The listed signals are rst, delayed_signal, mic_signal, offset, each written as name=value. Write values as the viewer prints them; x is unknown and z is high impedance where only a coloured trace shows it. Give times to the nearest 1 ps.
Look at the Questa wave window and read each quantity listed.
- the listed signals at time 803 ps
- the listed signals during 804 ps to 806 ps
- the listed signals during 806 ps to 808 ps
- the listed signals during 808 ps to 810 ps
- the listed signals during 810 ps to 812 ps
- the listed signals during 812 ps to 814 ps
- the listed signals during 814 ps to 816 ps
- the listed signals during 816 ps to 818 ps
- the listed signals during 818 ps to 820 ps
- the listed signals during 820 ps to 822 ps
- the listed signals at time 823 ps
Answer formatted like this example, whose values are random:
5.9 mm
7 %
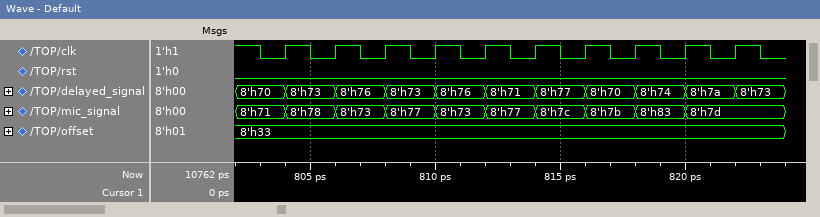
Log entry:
rst=0, delayed_signal=8'h70, mic_signal=8'h71, offset=8'h33
rst=0, delayed_signal=8'h73, mic_signal=8'h78, offset=8'h33
rst=0, delayed_signal=8'h76, mic_signal=8'h73, offset=8'h33
rst=0, delayed_signal=8'h73, mic_signal=8'h77, offset=8'h33
rst=0, delayed_signal=8'h76, mic_signal=8'h73, offset=8'h33
rst=0, delayed_signal=8'h71, mic_signal=8'h77, offset=8'h33
rst=0, delayed_signal=8'h77, mic_signal=8'h7c, offset=8'h33
rst=0, delayed_signal=8'h70, mic_signal=8'h7b, offset=8'h33
rst=0, delayed_signal=8'h74, mic_signal=8'h83, offset=8'h33
rst=0, delayed_signal=8'h7a, mic_signal=8'h7d, offset=8'h33
rst=0, delayed_signal=8'h73, mic_signal=8'h7d, offset=8'h33
